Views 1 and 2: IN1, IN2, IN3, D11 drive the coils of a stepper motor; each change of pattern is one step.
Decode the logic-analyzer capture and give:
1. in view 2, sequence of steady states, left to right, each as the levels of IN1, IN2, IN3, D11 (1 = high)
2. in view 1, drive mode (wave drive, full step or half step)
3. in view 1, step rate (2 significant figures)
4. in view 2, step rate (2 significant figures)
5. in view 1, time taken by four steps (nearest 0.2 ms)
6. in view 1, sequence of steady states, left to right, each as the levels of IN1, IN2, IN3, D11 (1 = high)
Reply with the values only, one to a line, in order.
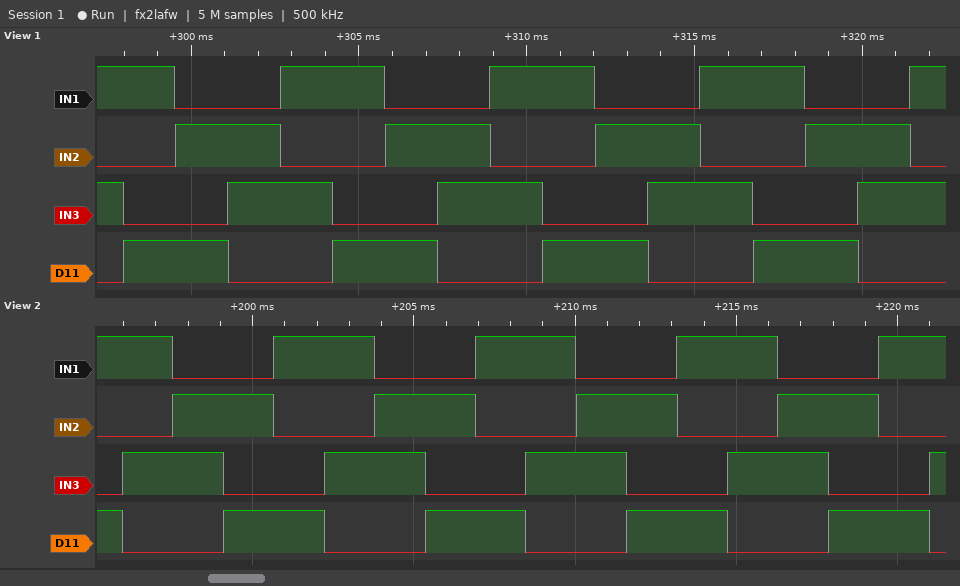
1001 1010 0110 0101 1001 1010 0110 0101 1001 1010 0110 0101 1001 1010 0110 0101 1001 1010
full step
640 steps/s
640 steps/s
6.2 ms
1010 1001 0101 0110 1010 1001 0101 0110 1010 1001 0101 0110 1010 1001 0101 0110 1010
